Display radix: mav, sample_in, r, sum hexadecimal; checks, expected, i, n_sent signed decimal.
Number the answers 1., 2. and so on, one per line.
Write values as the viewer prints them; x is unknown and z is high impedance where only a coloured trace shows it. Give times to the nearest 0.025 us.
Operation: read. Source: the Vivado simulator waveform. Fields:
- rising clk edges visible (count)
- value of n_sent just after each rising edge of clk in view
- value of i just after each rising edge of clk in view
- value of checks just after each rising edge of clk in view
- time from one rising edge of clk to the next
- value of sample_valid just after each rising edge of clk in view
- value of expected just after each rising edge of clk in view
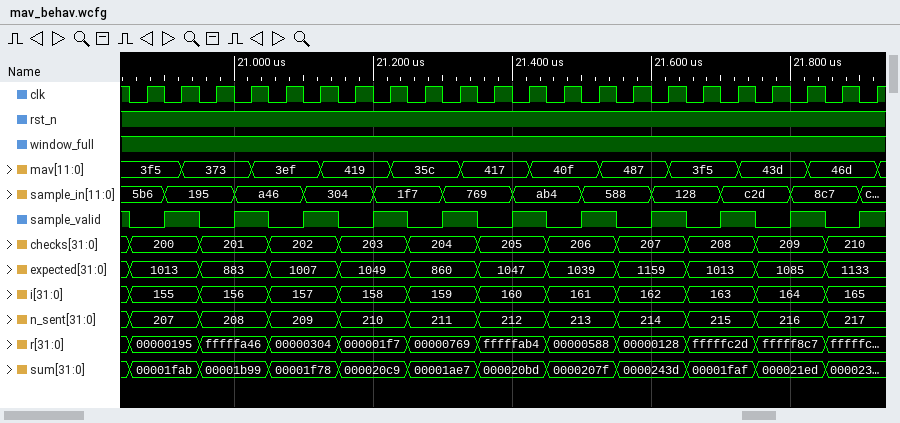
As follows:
1. 22
2. 207, 207, 208, 208, 209, 209, 210, 210, 211, 211, 212, 212, 213, 213, 214, 214, 215, 215, 216, 216, 217, 217
3. 155, 155, 156, 156, 157, 157, 158, 158, 159, 159, 160, 160, 161, 161, 162, 162, 163, 163, 164, 164, 165, 165
4. 200, 200, 201, 201, 202, 202, 203, 203, 204, 204, 205, 205, 206, 206, 207, 207, 208, 208, 209, 209, 210, 210
5. 0.05 us
6. 0 1 0 1 0 1 0 1 0 1 0 1 0 1 0 1 0 1 0 1 0 1
7. 1013, 1013, 883, 883, 1007, 1007, 1049, 1049, 860, 860, 1047, 1047, 1039, 1039, 1159, 1159, 1013, 1013, 1085, 1085, 1133, 1133
